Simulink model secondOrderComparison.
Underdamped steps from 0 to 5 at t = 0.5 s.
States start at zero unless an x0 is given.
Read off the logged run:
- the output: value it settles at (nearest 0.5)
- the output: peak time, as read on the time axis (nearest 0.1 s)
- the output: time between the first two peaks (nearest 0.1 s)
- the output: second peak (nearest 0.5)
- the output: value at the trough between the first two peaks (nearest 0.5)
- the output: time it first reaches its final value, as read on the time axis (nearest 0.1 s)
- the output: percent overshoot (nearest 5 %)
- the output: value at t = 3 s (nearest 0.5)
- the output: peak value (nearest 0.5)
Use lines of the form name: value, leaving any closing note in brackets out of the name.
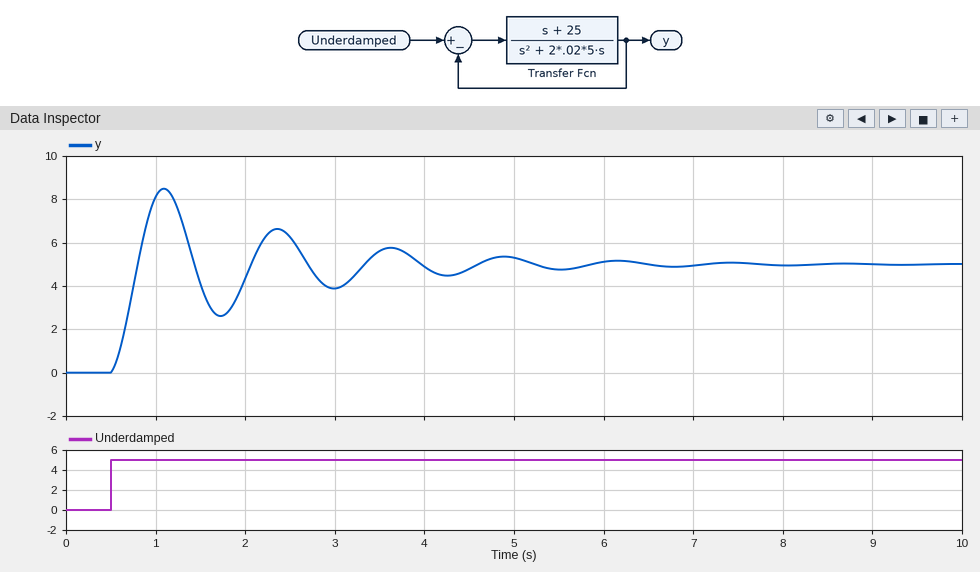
the output: value it settles at: 5.0
the output: peak time, as read on the time axis: 1.1 s
the output: time between the first two peaks: 1.3 s
the output: second peak: 6.5
the output: value at the trough between the first two peaks: 2.5
the output: time it first reaches its final value, as read on the time axis: 0.8 s
the output: percent overshoot: 70 %
the output: value at t = 3 s: 4.0
the output: peak value: 8.5
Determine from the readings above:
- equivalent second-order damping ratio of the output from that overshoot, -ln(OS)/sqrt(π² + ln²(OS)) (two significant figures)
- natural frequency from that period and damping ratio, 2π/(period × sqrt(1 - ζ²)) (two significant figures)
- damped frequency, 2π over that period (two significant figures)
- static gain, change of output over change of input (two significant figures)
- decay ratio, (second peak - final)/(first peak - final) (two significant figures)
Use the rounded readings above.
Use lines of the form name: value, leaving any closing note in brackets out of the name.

equivalent second-order damping ratio of the output from that overshoot, -ln(OS)/sqrt(π² + ln²(OS)): 0.11
natural frequency from that period and damping ratio, 2π/(period × sqrt(1 - ζ²)): 4.9 rad/s
damped frequency, 2π over that period: 4.8 rad/s
static gain, change of output over change of input: 1.0
decay ratio, (second peak - final)/(first peak - final): 0.43
